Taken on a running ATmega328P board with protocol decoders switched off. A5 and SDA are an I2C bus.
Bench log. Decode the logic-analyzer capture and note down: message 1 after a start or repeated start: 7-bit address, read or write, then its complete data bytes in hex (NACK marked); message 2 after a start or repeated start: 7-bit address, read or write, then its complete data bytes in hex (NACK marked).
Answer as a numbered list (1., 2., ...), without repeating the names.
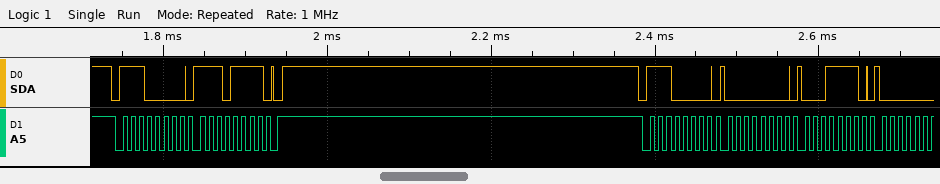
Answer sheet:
1. 0x70 write: EF
2. 0x70 write: 00 1E
